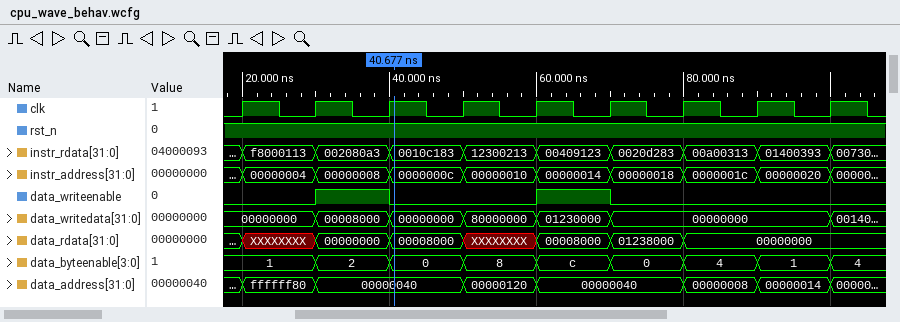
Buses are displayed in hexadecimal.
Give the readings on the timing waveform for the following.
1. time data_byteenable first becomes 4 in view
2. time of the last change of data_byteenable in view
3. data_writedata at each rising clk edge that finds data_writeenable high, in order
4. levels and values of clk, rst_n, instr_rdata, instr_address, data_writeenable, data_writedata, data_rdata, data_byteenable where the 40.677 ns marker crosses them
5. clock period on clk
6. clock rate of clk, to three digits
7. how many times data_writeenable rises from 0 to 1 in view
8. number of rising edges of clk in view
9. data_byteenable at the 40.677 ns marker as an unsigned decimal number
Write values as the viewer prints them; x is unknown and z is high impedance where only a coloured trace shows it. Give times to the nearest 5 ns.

80 ns
100 ns
00008000, 01230000
clk=1, rst_n=1, instr_rdata=0010c183, instr_address=0000000c, data_writeenable=0, data_writedata=00000000, data_rdata=00008000, data_byteenable=0
10 ns
100 MHz
2
9
0
